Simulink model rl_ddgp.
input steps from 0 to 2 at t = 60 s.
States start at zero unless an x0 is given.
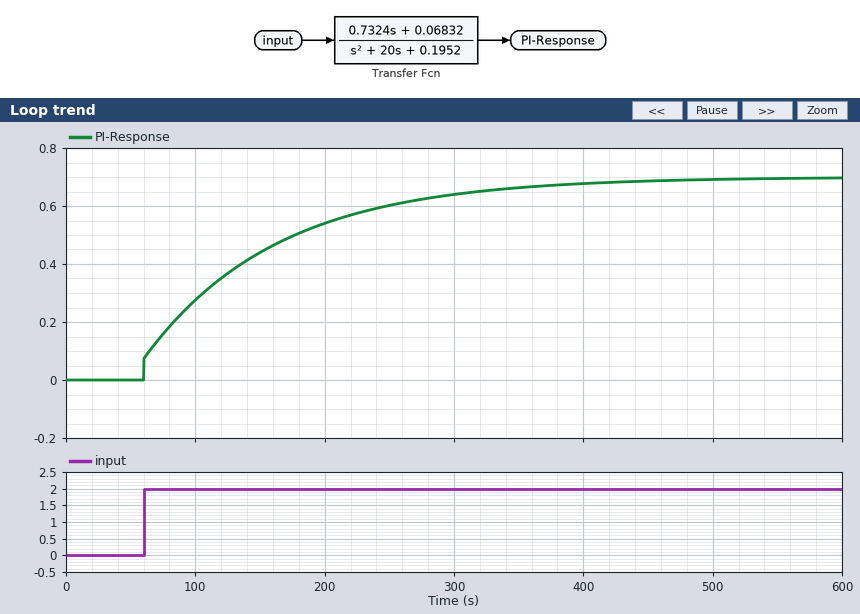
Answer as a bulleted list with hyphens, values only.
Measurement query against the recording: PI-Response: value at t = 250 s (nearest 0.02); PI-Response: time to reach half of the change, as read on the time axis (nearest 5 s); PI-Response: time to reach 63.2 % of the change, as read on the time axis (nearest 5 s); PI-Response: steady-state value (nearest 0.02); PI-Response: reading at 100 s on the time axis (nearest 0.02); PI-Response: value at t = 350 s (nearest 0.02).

- 0.60
- 120 s
- 150 s
- 0.70
- 0.28
- 0.66
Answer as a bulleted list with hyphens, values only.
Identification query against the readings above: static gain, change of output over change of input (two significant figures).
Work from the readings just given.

- 0.35
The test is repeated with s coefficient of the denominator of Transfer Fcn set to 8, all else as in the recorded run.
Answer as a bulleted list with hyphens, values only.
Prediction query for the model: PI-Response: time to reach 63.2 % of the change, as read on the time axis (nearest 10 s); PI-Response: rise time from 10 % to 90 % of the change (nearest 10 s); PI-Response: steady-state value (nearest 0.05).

- 90 s
- 80 s
- 0.70
